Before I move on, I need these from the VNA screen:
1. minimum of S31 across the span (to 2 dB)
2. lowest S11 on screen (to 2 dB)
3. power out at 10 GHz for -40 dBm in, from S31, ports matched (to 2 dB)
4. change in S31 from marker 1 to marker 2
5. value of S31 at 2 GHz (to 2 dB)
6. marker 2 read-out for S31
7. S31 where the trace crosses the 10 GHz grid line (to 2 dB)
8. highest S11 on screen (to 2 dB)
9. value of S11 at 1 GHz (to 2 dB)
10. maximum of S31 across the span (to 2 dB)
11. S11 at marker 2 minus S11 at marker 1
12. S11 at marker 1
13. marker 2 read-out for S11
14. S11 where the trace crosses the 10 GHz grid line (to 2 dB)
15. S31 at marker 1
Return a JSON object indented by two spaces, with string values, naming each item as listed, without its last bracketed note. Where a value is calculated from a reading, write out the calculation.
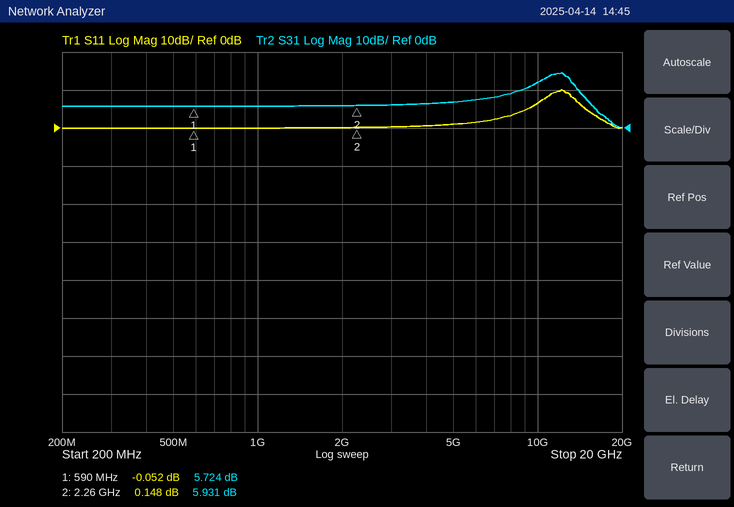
{
  "minimum of S31 across the span": "0 dB",
  "lowest S11 on screen": "0 dB",
  "power out at 10 GHz for -40 dBm in, from S31, ports matched": "-40 dBm + (12 dB) = -28 dBm",
  "change in S31 from marker 1 to marker 2": "5.931 − (5.724) = 0.207 dB",
  "value of S31 at 2 GHz": "6 dB",
  "marker 2 read-out for S31": "5.931 dB",
  "S31 where the trace crosses the 10 GHz grid line": "12 dB",
  "highest S11 on screen": "10 dB",
  "value of S11 at 1 GHz": "0 dB",
  "maximum of S31 across the span": "14 dB",
  "S11 at marker 2 minus S11 at marker 1": "0.148 − (-0.052) = 0.200 dB",
  "S11 at marker 1": "-0.052 dB",
  "marker 2 read-out for S11": "0.148 dB",
  "S11 where the trace crosses the 10 GHz grid line": "6 dB",
  "S31 at marker 1": "5.724 dB"
}
